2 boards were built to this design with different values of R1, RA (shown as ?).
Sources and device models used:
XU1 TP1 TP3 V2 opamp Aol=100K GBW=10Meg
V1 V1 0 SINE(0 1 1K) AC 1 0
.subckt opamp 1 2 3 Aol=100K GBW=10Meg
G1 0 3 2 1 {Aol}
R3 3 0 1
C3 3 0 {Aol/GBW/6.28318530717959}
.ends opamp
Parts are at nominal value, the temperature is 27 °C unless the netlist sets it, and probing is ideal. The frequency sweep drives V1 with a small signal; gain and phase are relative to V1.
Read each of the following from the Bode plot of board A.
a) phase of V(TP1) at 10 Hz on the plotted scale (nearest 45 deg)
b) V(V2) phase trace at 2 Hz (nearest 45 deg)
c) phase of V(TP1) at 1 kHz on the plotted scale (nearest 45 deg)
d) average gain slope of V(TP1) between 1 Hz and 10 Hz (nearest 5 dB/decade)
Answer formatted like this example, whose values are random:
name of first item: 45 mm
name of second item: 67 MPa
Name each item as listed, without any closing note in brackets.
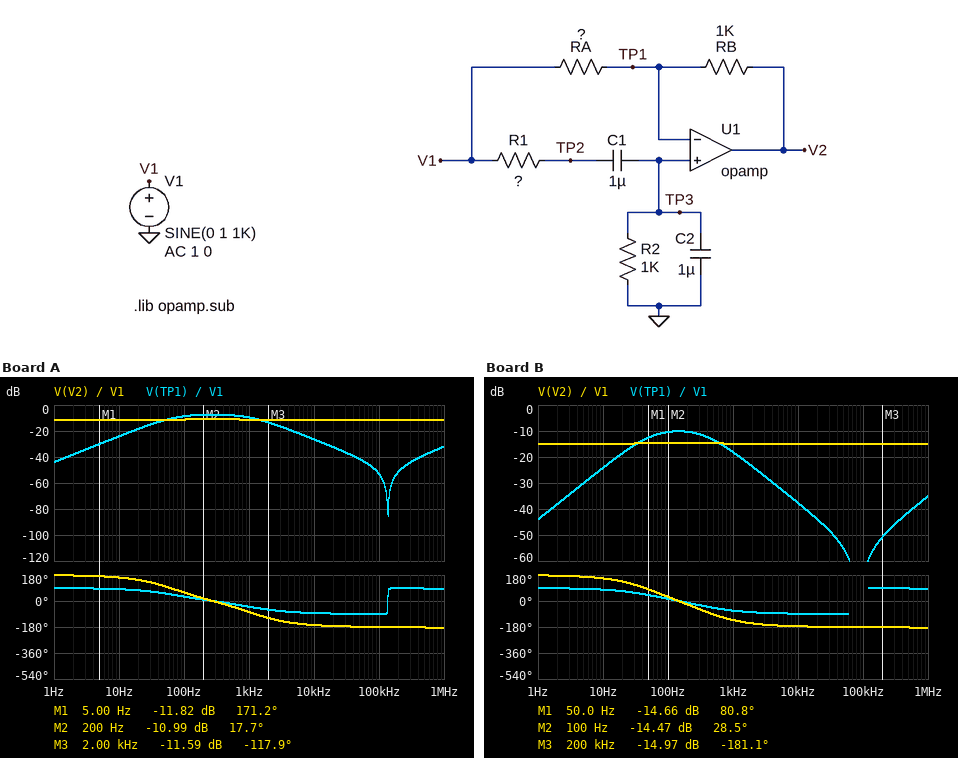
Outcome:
phase of V(TP1) at 10 Hz on the plotted scale: 90 deg
V(V2) phase trace at 2 Hz: 180 deg
phase of V(TP1) at 1 kHz on the plotted scale: -45 deg
average gain slope of V(TP1) between 1 Hz and 10 Hz: 20 dB/decade
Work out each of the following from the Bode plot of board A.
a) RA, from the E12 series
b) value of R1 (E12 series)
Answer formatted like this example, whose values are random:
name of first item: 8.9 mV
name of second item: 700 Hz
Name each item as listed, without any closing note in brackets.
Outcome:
RA, from the E12 series: 3.9 kΩ
value of R1: 330 Ω
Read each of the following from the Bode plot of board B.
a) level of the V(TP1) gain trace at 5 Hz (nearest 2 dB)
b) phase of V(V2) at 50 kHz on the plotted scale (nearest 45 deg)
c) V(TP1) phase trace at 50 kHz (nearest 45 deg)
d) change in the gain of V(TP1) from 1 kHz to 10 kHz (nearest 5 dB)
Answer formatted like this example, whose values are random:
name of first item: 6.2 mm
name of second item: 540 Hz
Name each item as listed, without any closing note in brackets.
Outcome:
level of the V(TP1) gain trace at 5 Hz: -30 dB
phase of V(V2) at 50 kHz on the plotted scale: -180 deg
V(TP1) phase trace at 50 kHz: -90 deg
change in the gain of V(TP1) from 1 kHz to 10 kHz: -20 dB
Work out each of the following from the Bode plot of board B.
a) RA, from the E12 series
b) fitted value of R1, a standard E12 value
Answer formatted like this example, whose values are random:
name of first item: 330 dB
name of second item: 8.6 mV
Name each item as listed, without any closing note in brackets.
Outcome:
RA, from the E12 series: 5.6 kΩ
fitted value of R1, a standard E12 value: 1.2 kΩ
